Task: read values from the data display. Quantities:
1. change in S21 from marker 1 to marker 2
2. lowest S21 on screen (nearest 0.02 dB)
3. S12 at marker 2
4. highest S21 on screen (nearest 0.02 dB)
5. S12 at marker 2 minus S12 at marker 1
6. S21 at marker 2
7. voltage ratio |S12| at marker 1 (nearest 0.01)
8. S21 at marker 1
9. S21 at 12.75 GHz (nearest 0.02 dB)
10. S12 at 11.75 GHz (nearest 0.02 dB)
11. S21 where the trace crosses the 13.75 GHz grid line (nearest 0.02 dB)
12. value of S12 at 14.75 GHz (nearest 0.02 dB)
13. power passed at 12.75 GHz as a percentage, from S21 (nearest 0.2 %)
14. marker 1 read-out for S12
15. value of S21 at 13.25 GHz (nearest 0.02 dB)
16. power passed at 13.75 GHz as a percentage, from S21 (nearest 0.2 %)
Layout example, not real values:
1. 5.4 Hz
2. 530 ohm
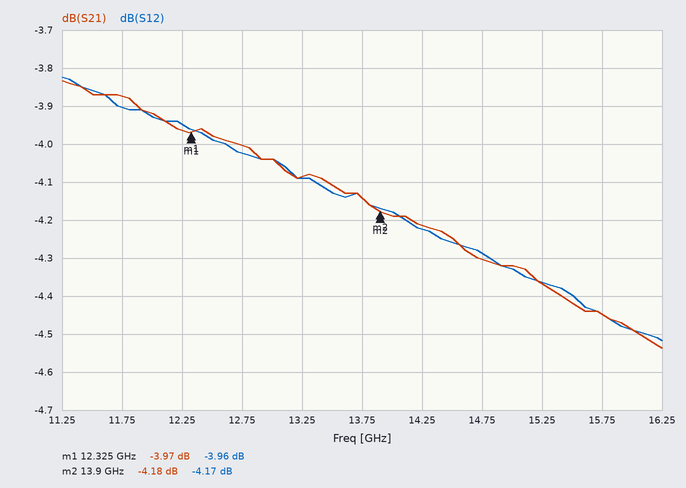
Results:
1. -0.21 dB
2. -4.54 dB
3. -4.17 dB
4. -3.84 dB
5. -0.21 dB
6. -4.18 dB
7. 0.63
8. -3.97 dB
9. -4.00 dB
10. -3.90 dB
11. -4.14 dB
12. -4.28 dB
13. 39.8 %
14. -3.96 dB
15. -4.08 dB
16. 38.6 %
